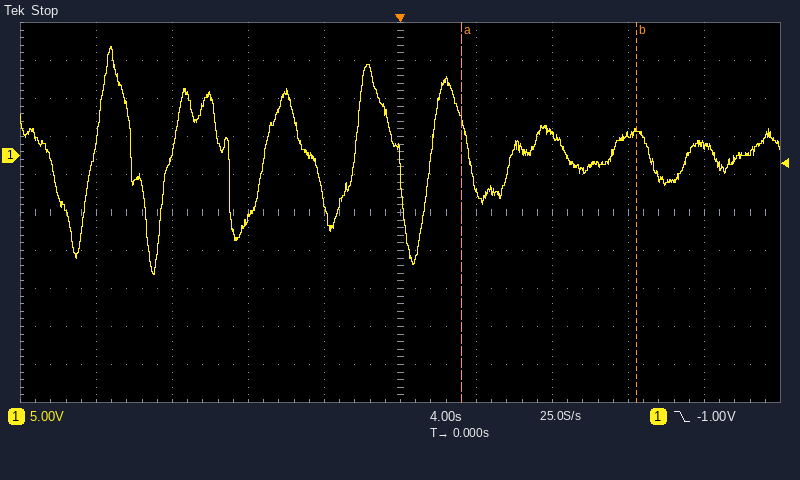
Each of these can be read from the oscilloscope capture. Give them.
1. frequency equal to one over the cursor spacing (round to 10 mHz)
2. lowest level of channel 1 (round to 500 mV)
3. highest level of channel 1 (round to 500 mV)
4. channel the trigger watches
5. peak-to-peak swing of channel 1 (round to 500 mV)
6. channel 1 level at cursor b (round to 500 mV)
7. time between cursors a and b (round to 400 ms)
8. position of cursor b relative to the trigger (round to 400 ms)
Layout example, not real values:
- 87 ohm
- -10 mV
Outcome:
- 110 mHz
- -15.5 V
- 14.5 V
- channel 1
- 30.0 V
- 3.0 V
- 9.2 s
- +12.4 s
